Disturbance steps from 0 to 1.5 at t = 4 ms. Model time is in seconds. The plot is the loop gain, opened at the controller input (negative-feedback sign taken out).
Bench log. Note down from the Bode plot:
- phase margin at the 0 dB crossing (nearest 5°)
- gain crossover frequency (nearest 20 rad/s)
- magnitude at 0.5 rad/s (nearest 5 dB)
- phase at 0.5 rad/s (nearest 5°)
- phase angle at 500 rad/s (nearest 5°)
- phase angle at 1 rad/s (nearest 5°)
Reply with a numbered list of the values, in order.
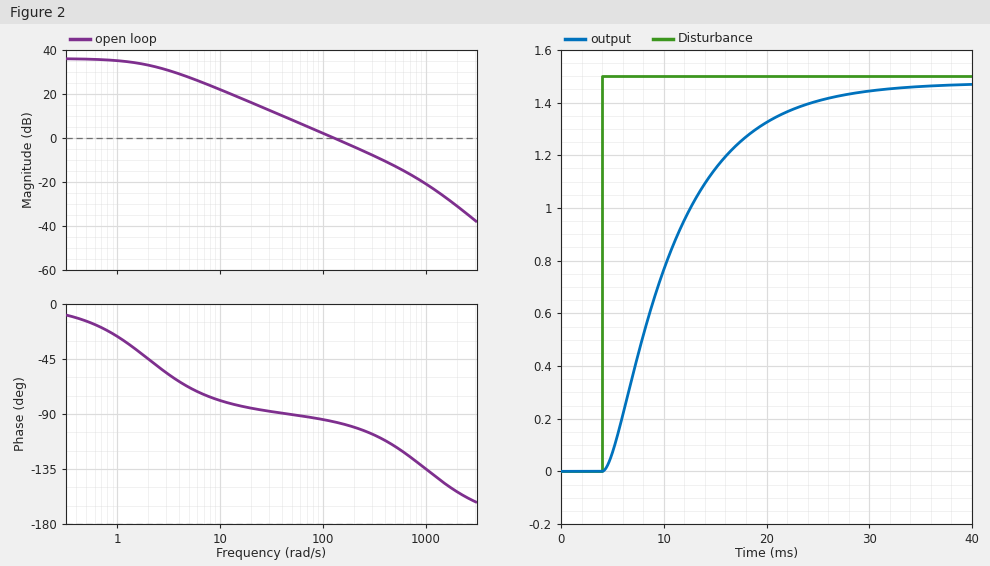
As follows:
1. 85°
2. 120 rad/s
3. 35 dB
4. -15°
5. -115°
6. -25°
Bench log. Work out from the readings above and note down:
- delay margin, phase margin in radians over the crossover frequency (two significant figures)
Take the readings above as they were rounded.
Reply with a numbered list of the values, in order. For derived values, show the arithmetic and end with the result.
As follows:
1. 85 × π / 180 / 120 = 0.012 s
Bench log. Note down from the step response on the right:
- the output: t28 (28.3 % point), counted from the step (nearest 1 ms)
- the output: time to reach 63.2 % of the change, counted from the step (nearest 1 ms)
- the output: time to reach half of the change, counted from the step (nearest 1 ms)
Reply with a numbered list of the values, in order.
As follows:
1. 3 ms
2. 8 ms
3. 6 ms
